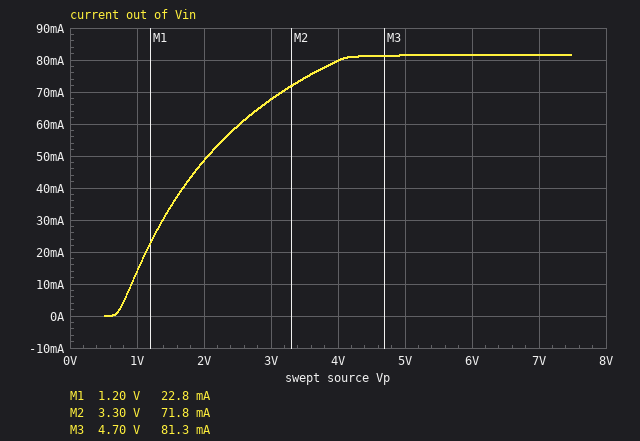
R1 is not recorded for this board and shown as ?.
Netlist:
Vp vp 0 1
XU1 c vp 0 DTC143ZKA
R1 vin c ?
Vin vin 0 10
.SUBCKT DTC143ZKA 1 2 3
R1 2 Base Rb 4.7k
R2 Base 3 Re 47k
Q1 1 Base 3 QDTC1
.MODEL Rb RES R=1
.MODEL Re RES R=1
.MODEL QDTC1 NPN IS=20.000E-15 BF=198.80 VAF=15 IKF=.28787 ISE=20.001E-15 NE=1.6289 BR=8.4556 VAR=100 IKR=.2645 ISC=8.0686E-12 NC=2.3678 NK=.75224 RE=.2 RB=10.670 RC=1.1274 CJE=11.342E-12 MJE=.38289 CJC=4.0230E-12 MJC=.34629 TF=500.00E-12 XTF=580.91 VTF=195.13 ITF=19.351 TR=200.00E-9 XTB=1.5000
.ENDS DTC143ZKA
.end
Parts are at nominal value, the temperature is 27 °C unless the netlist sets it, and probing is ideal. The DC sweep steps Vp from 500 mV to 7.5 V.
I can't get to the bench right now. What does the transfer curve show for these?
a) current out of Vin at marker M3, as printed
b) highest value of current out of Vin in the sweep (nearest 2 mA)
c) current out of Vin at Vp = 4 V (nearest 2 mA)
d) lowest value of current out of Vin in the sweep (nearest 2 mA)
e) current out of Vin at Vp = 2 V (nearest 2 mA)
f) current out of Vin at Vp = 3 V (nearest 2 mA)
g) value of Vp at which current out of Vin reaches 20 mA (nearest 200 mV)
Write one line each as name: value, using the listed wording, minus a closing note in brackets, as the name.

current out of Vin at marker M3, as printed: 81.3 mA
highest value of current out of Vin in the sweep: 82 mA
current out of Vin at Vp = 4 V: 80 mA
lowest value of current out of Vin in the sweep: 0 A
current out of Vin at Vp = 2 V: 48 mA
current out of Vin at Vp = 3 V: 68 mA
value of Vp at which current out of Vin reaches 20 mA: 1.2 V
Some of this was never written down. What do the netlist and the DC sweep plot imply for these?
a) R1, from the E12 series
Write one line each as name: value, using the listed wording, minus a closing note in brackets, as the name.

R1, from the E12 series: 120 Ω
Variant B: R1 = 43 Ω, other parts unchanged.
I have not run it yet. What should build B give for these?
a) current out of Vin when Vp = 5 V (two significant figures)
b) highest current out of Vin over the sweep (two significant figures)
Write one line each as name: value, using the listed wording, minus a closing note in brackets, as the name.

current out of Vin when Vp = 5 V: 120 mA
highest current out of Vin over the sweep: 150 mA
